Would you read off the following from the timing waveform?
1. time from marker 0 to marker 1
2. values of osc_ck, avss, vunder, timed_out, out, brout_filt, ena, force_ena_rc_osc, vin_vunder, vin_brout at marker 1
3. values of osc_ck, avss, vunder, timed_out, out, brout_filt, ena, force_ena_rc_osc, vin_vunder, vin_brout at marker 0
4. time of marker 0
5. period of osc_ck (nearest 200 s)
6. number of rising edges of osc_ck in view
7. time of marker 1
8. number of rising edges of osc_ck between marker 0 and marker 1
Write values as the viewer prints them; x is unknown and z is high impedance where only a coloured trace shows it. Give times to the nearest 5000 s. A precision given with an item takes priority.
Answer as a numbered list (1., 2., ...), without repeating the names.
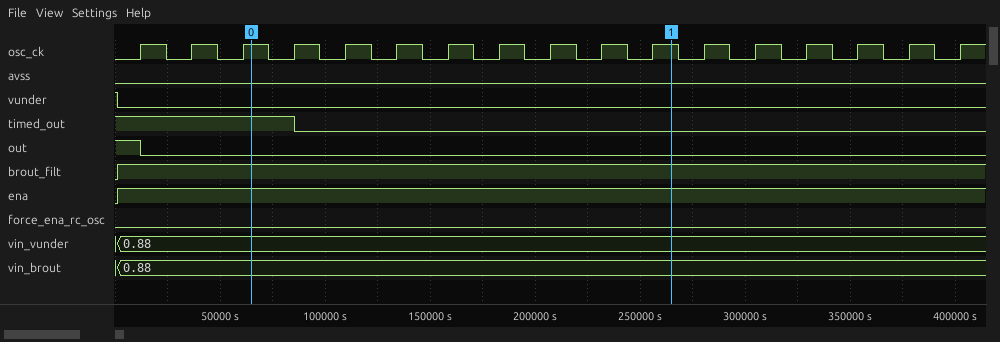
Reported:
1. 200000 s
2. osc_ck=1, avss=0, vunder=0, timed_out=0, out=0, brout_filt=1, ena=1, force_ena_rc_osc=0, vin_vunder=0.88, vin_brout=0.88
3. osc_ck=1, avss=0, vunder=0, timed_out=1, out=0, brout_filt=1, ena=1, force_ena_rc_osc=0, vin_vunder=0.88, vin_brout=0.88
4. 65000 s
5. 24400 s
6. 17
7. 265000 s
8. 8
